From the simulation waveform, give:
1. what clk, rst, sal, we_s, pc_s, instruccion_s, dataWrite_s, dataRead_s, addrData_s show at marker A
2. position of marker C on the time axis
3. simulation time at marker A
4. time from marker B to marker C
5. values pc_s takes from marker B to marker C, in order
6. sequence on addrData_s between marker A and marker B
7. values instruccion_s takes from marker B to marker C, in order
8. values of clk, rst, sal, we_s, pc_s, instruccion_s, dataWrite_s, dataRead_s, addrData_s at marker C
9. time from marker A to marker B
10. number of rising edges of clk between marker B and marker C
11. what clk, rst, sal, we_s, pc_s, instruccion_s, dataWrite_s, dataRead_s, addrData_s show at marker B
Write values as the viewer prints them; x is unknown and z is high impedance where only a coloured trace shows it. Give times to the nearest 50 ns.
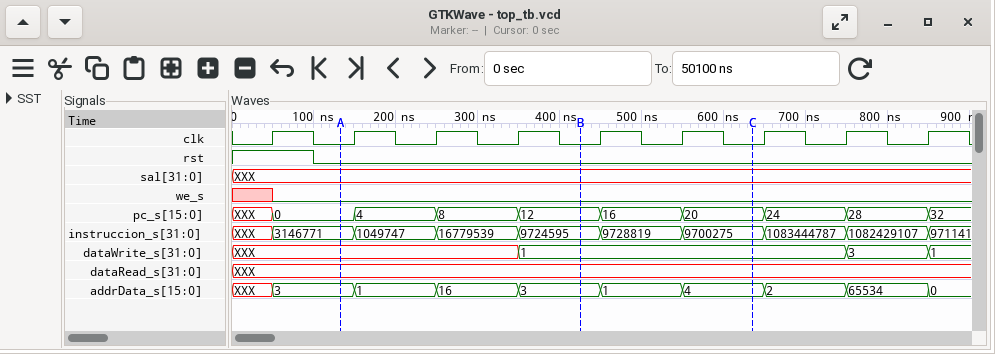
clk=0, rst=0, sal=XXX, we_s=0, pc_s=0, instruccion_s=3146771, dataWrite_s=XXX, dataRead_s=XXX, addrData_s=3
650 ns
150 ns
200 ns
12, 16, 20
3, 1, 16, 3
9724595, 9728819, 9700275
clk=0, rst=0, sal=XXX, we_s=0, pc_s=20, instruccion_s=9700275, dataWrite_s=1, dataRead_s=XXX, addrData_s=4
300 ns
2
clk=0, rst=0, sal=XXX, we_s=0, pc_s=12, instruccion_s=9724595, dataWrite_s=1, dataRead_s=XXX, addrData_s=3
